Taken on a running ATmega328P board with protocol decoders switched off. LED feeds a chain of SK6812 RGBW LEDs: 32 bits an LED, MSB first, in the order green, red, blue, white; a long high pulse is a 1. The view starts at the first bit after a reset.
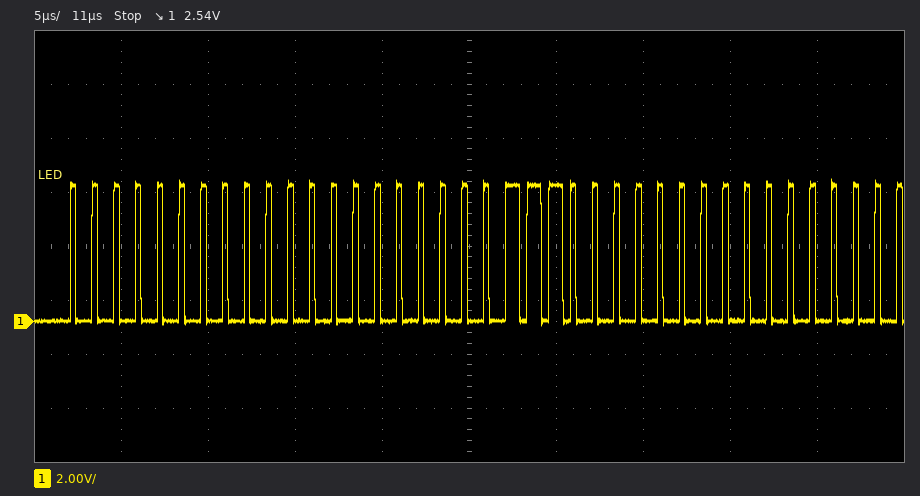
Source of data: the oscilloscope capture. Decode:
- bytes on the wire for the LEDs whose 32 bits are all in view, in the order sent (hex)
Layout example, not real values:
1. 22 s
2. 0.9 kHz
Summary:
1. 00 00 0E 00
